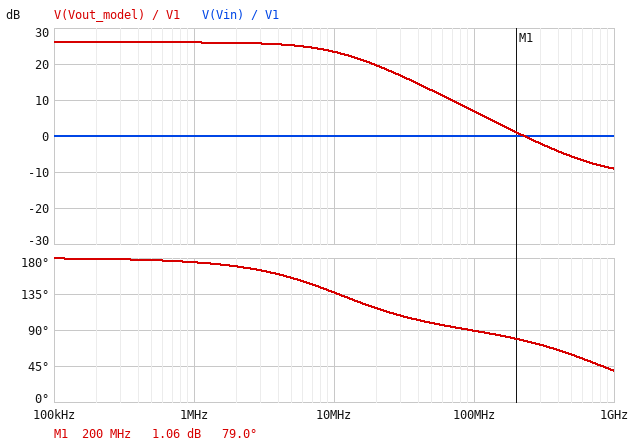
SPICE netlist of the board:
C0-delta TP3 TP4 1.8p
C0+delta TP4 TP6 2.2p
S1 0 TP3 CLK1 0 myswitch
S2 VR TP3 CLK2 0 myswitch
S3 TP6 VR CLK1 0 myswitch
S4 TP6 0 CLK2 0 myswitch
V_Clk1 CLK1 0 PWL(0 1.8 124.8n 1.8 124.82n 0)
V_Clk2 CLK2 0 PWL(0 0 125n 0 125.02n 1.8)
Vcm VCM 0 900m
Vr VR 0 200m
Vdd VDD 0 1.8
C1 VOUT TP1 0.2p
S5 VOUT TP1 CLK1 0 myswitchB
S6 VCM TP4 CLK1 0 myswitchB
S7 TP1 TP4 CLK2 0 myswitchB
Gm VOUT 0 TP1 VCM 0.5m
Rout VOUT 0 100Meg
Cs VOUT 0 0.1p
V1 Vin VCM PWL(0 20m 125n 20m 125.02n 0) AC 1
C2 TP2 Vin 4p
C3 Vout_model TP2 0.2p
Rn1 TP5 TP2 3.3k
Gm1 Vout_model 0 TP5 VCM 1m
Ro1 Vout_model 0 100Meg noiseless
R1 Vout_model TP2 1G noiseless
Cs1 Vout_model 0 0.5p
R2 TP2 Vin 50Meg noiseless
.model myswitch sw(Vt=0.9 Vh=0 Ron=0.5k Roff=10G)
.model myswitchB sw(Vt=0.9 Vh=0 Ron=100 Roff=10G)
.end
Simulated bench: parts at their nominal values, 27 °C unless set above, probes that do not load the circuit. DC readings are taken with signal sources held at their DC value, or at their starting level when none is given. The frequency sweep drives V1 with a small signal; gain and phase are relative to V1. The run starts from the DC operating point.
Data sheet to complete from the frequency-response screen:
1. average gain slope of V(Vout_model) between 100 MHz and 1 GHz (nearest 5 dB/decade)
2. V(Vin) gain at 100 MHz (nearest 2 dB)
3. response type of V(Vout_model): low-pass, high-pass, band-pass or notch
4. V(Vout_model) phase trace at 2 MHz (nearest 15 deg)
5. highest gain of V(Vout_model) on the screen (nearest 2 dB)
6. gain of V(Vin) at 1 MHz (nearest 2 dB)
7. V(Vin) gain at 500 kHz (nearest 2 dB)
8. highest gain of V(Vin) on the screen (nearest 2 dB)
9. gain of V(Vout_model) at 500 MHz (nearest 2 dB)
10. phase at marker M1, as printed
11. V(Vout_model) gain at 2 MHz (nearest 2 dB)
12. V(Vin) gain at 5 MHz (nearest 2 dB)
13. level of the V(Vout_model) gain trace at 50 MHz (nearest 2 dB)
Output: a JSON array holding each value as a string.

["-15 dB/decade", "0 dB", "low-pass", "165 deg", "26 dB", "0 dB", "0 dB", "0 dB", "-6 dB", "79.0 deg", "26 dB", "0 dB", "12 dB"]
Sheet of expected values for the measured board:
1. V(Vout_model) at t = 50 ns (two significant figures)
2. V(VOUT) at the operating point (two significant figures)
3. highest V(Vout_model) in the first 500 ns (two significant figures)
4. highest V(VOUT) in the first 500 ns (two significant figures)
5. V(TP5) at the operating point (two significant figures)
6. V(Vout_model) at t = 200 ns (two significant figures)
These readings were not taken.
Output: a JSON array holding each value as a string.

["500 mV", "900 mV", "900 mV", "1.3 V", "900 mV", "900 mV"]
